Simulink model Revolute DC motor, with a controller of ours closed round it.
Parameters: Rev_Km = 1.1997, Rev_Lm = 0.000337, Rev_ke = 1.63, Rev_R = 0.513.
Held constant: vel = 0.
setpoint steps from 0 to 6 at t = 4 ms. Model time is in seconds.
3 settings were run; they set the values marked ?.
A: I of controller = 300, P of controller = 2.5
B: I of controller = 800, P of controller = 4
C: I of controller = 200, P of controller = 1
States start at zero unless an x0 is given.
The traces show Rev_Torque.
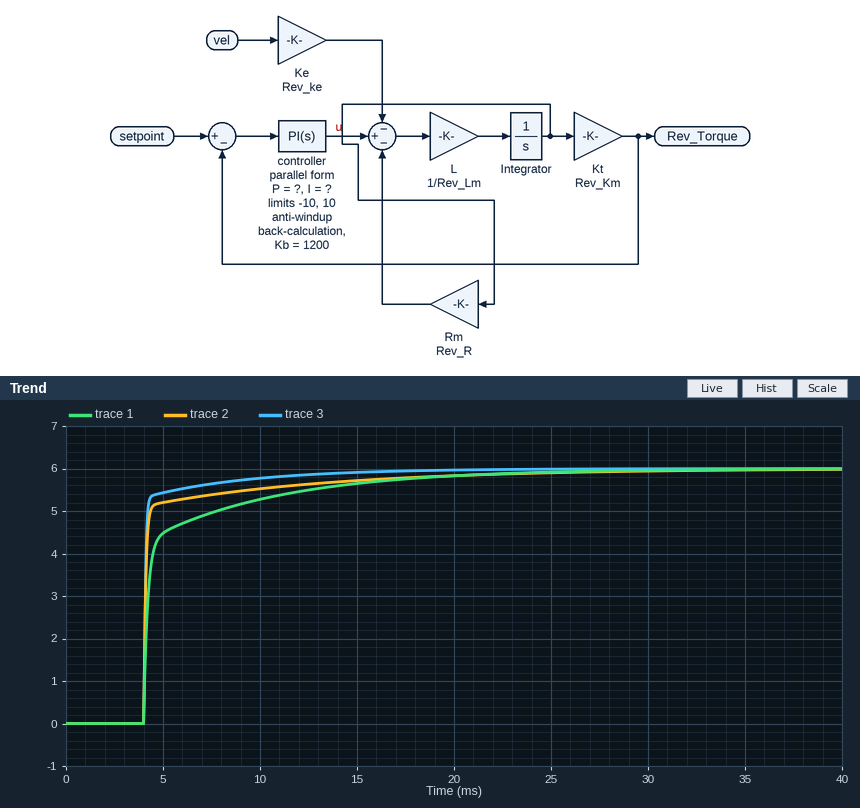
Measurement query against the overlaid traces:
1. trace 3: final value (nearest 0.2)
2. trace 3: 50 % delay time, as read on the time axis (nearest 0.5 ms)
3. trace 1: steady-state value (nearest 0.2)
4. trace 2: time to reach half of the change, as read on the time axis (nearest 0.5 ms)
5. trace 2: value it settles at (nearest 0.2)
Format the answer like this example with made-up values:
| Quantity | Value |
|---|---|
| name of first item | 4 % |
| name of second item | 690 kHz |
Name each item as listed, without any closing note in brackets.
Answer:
| Quantity | Value |
|---|---|
| trace 3: final value | 6.0 |
| trace 3: 50 % delay time, as read on the time axis | 4.0 ms |
| trace 1: steady-state value | 6.0 |
| trace 2: time to reach half of the change, as read on the time axis | 4.0 ms |
| trace 2: value it settles at | 6.0 |
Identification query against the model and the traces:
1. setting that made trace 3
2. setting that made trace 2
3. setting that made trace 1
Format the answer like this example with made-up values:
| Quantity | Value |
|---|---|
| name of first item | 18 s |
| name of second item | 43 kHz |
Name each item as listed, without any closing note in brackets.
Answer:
| Quantity | Value |
|---|---|
| setting that made trace 3 | B |
| setting that made trace 2 | A |
| setting that made trace 1 | C |
